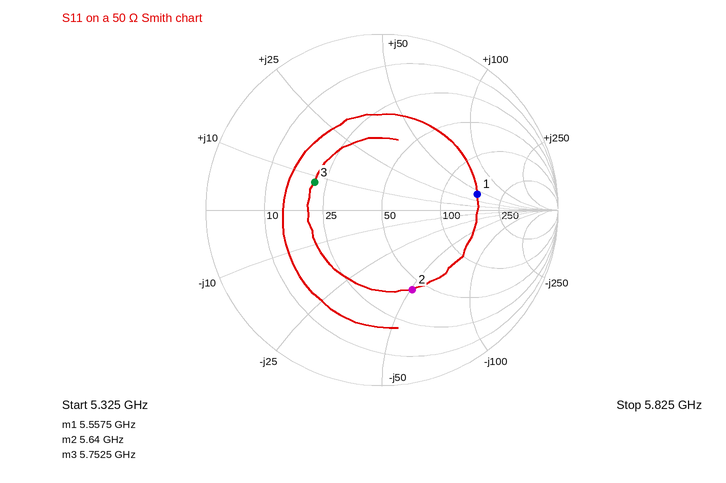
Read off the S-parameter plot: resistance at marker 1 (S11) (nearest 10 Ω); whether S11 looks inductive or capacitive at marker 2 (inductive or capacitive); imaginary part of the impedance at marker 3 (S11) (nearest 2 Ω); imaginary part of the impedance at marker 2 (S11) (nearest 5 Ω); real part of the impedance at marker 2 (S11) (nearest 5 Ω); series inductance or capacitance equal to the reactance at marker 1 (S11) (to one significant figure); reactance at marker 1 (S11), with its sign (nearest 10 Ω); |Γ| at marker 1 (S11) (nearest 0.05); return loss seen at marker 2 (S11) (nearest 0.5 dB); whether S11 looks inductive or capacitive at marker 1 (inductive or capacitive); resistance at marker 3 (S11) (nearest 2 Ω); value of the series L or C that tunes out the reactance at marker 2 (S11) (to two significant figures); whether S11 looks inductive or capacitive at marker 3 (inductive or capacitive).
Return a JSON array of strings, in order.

["160 Ω", "capacitive", "+8 Ω", "-50 Ω", "45 Ω", "1 nH", "+40 Ω", "0.55", "6.5 dB", "inductive", "22 Ω", "1.4 nH", "inductive"]
